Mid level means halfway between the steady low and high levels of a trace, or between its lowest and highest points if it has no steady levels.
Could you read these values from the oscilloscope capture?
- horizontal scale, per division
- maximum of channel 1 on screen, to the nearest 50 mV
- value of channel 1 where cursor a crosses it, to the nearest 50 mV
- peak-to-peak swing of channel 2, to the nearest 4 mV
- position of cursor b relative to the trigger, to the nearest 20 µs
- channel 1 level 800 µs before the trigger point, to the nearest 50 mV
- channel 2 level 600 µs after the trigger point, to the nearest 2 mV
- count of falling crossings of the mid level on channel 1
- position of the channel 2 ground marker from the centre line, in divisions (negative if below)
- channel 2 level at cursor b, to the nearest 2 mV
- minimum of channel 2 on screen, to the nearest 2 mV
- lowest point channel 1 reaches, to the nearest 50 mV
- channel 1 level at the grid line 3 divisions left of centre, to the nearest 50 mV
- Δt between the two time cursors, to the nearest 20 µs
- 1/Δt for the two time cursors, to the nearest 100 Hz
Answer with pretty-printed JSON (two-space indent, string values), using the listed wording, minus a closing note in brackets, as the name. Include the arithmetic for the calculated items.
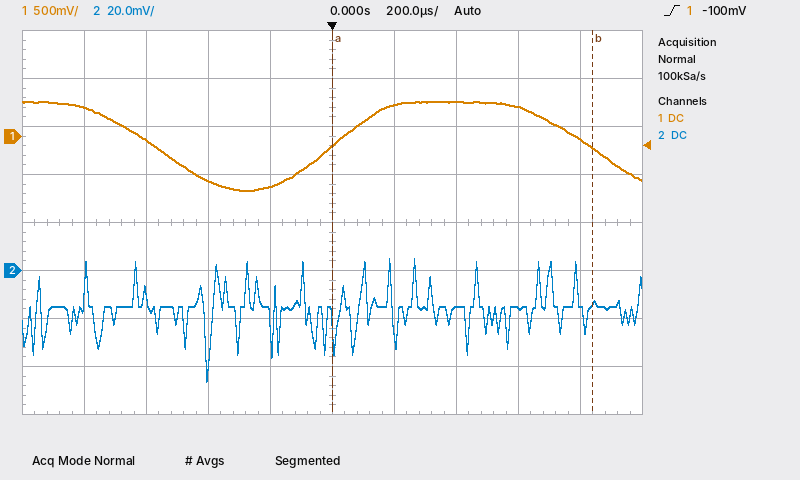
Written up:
{
  "horizontal scale, per division": "200 µs",
  "maximum of channel 1 on screen, to the nearest 50 mV": "350 mV",
  "value of channel 1 where cursor a crosses it, to the nearest 50 mV": "-100 mV",
  "peak-to-peak swing of channel 2, to the nearest 4 mV": "52 mV",
  "position of cursor b relative to the trigger, to the nearest 20 µs": "+840 µs",
  "channel 1 level 800 µs before the trigger point, to the nearest 50 mV": "300 mV",
  "channel 2 level 600 µs after the trigger point, to the nearest 2 mV": "-16 mV",
  "count of falling crossings of the mid level on channel 1": "2",
  "position of the channel 2 ground marker from the centre line, in divisions": "-1.0 div",
  "channel 2 level at cursor b, to the nearest 2 mV": "-14 mV",
  "minimum of channel 2 on screen, to the nearest 2 mV": "-46 mV",
  "lowest point channel 1 reaches, to the nearest 50 mV": "-550 mV",
  "channel 1 level at the grid line 3 divisions left of centre, to the nearest 50 mV": "-50 mV",
  "Δt between the two time cursors, to the nearest 20 µs": "840 µs",
  "1/Δt for the two time cursors, to the nearest 100 Hz": "1 / 840 µs ≈ 1.2 kHz"
}
